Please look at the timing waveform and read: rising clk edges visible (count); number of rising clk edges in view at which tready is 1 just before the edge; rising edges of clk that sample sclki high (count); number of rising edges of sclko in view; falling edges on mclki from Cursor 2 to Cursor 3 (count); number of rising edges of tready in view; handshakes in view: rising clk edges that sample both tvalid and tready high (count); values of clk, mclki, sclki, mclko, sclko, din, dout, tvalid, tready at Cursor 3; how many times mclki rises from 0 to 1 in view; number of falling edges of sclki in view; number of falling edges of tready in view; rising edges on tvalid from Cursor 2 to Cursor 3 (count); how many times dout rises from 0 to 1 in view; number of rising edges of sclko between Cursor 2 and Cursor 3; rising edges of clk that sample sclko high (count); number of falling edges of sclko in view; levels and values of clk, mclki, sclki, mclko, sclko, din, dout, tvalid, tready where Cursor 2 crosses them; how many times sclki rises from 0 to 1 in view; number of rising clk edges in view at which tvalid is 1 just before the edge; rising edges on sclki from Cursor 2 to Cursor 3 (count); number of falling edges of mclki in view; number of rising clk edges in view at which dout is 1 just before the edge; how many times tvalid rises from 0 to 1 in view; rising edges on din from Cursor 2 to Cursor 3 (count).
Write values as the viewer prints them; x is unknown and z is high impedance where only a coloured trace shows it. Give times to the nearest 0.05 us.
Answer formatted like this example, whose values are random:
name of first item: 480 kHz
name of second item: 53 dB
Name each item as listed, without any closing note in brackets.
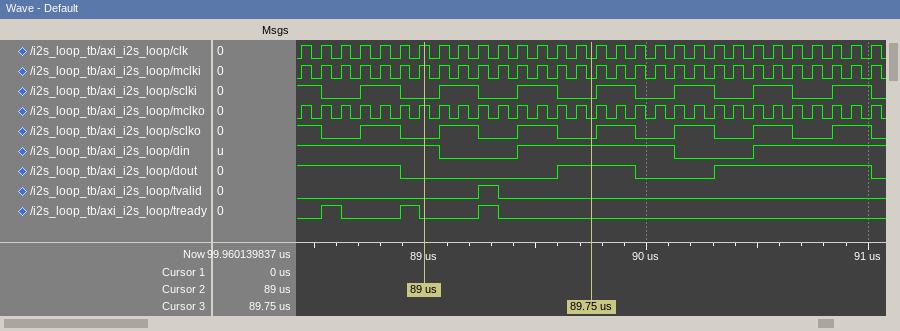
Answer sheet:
rising clk edges visible: 30
number of rising clk edges in view at which tready is 1 just before the edge: 3
rising edges of clk that sample sclki high: 16
number of rising edges of sclko in view: 7
falling edges on mclki from Cursor 2 to Cursor 3: 9
number of rising edges of tready in view: 3
handshakes in view: rising clk edges that sample both tvalid and tready high: 1
values of clk, mclki, sclki, mclko, sclko, din, dout, tvalid, tready at Cursor 3: clk=0, mclki=0, sclki=0, mclko=0, sclko=0, din=1, dout=1, tvalid=0, tready=0
how many times mclki rises from 0 to 1 in view: 30
number of falling edges of sclki in view: 8
number of falling edges of tready in view: 3
rising edges on tvalid from Cursor 2 to Cursor 3: 1
how many times dout rises from 0 to 1 in view: 2
number of rising edges of sclko between Cursor 2 and Cursor 3: 2
rising edges of clk that sample sclko high: 16
number of falling edges of sclko in view: 8
levels and values of clk, mclki, sclki, mclko, sclko, din, dout, tvalid, tready where Cursor 2 crosses them: clk=1, mclki=1, sclki=0, mclko=1, sclko=0, din=1, dout=0, tvalid=0, tready=0
how many times sclki rises from 0 to 1 in view: 7
number of rising clk edges in view at which tvalid is 1 just before the edge: 1
rising edges on sclki from Cursor 2 to Cursor 3: 2
number of falling edges of mclki in view: 30
number of rising clk edges in view at which dout is 1 just before the edge: 18
how many times tvalid rises from 0 to 1 in view: 1
rising edges on din from Cursor 2 to Cursor 3: 1
